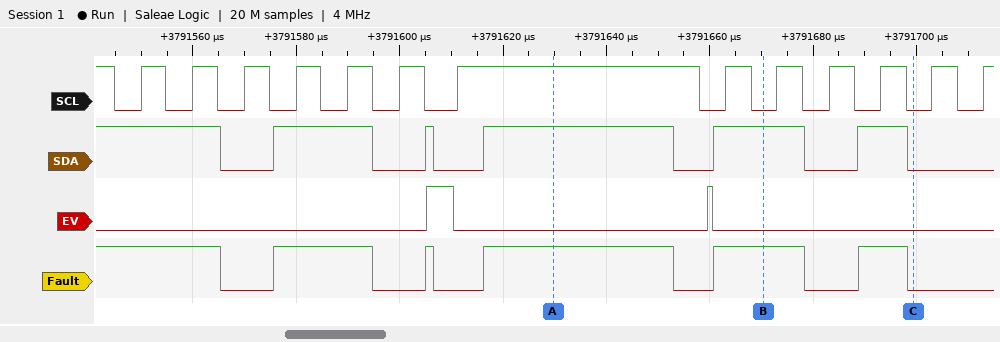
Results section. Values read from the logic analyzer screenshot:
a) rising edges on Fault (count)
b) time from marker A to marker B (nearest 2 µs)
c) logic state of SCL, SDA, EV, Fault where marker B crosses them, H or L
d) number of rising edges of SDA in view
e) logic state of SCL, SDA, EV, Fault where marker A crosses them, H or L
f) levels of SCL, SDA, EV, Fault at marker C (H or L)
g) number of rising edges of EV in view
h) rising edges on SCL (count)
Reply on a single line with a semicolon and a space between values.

5; 40 µs; SCL=L, SDA=H, EV=L, Fault=H; 5; SCL=H, SDA=H, EV=L, Fault=H; SCL=L, SDA=L, EV=L, Fault=L; 2; 13
